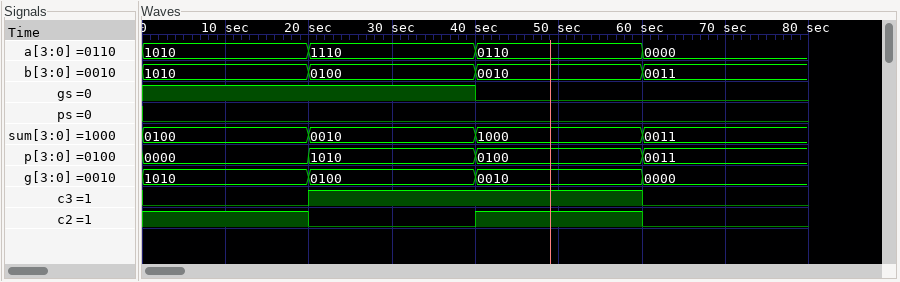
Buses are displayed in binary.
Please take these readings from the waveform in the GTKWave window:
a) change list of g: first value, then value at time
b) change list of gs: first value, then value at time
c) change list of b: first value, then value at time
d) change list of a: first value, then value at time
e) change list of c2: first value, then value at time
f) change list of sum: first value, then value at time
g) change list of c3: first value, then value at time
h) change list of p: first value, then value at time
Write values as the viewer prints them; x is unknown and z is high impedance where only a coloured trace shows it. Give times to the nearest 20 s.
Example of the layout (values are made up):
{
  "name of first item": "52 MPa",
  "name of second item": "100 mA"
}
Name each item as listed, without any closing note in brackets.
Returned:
{
  "change list of g: first value, then value at time": "1010, 0100 at 20 s, 0010 at 40 s, 0000 at 60 s",
  "change list of gs: first value, then value at time": "1, 0 at 40 s",
  "change list of b: first value, then value at time": "1010, 0100 at 20 s, 0010 at 40 s, 0011 at 60 s",
  "change list of a: first value, then value at time": "1010, 1110 at 20 s, 0110 at 40 s, 0000 at 60 s",
  "change list of c2: first value, then value at time": "1, 0 at 20 s, 1 at 40 s, 0 at 60 s",
  "change list of sum: first value, then value at time": "0100, 0010 at 20 s, 1000 at 40 s, 0011 at 60 s",
  "change list of c3: first value, then value at time": "0, 1 at 20 s, 0 at 60 s",
  "change list of p: first value, then value at time": "0000, 1010 at 20 s, 0100 at 40 s, 0011 at 60 s"
}
